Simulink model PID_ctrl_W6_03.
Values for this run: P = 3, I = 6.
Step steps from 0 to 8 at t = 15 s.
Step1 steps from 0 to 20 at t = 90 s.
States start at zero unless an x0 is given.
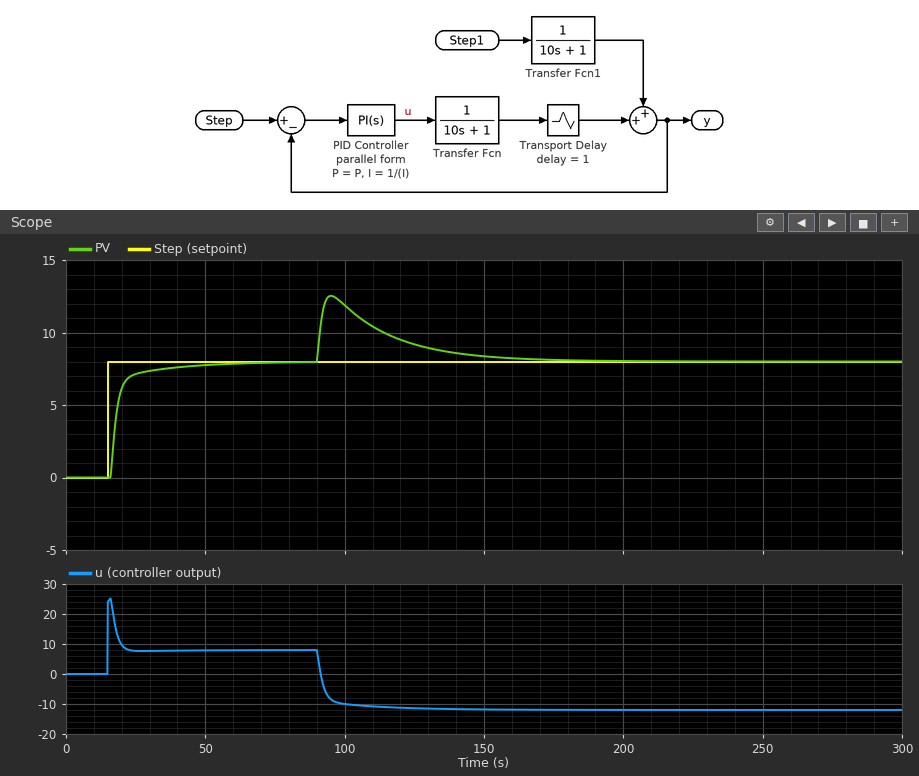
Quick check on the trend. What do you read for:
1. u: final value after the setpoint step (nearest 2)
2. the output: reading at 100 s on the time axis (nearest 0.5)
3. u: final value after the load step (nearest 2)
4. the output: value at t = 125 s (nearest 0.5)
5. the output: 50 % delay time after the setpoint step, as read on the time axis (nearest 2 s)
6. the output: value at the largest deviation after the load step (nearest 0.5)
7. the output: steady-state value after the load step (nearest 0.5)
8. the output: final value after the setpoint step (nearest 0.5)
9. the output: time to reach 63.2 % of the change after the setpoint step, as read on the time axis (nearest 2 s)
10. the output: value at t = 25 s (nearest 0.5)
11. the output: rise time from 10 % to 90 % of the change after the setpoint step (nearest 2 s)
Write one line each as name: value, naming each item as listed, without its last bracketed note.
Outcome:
u: final value after the setpoint step: 8
the output: reading at 100 s on the time axis: 12.0
u: final value after the load step: -12
the output: value at t = 125 s: 9.0
the output: 50 % delay time after the setpoint step, as read on the time axis: 18 s
the output: value at the largest deviation after the load step: 12.5
the output: steady-state value after the load step: 8.0
the output: final value after the setpoint step: 8.0
the output: time to reach 63.2 % of the change after the setpoint step, as read on the time axis: 18 s
the output: value at t = 25 s: 7.0
the output: rise time from 10 % to 90 % of the change after the setpoint step: 10 s
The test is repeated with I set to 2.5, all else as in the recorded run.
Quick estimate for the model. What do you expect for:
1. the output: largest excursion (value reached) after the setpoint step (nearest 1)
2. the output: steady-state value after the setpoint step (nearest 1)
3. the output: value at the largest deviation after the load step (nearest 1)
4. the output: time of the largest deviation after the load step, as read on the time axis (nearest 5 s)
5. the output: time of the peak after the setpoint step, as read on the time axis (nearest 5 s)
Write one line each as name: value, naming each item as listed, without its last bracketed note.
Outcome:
the output: largest excursion (value reached) after the setpoint step: 8
the output: steady-state value after the setpoint step: 8
the output: value at the largest deviation after the load step: 12
the output: time of the largest deviation after the load step, as read on the time axis: 95 s
the output: time of the peak after the setpoint step, as read on the time axis: 25 s
